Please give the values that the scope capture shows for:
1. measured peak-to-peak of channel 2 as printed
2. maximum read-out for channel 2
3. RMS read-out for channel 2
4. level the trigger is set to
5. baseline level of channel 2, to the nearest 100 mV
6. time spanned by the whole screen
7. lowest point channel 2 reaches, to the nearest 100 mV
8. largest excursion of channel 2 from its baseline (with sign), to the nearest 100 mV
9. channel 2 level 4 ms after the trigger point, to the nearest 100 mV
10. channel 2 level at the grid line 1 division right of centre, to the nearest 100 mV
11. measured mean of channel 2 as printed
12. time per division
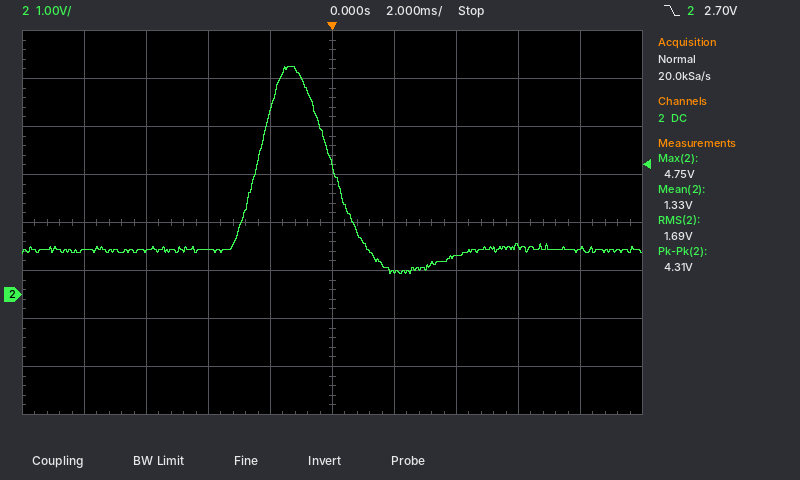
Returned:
4.31 V
4.75 V
1.69 V
2.70 V
900 mV
20 ms
400 mV
+3.8 V
800 mV
500 mV
1.33 V
2 ms
